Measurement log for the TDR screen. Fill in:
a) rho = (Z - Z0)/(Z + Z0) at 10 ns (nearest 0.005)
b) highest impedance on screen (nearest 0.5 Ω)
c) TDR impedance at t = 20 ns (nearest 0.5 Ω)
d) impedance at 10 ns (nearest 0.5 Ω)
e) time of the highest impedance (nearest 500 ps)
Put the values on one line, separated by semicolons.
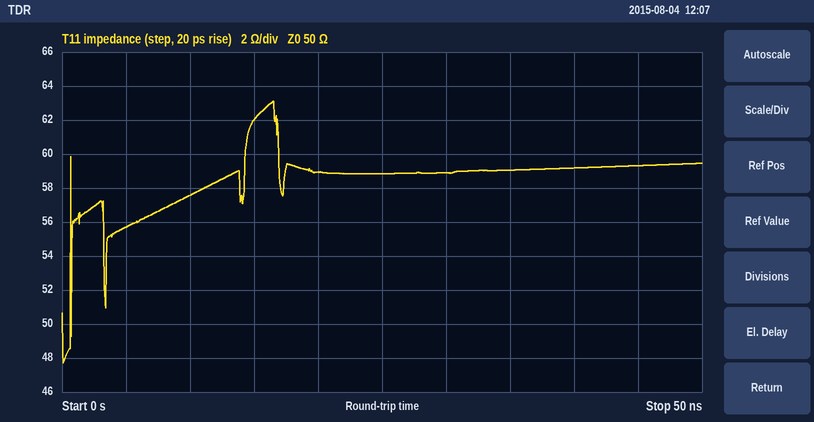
+0.070; 63.0 Ω; 59.0 Ω; 57.5 Ω; 16.5 ns
